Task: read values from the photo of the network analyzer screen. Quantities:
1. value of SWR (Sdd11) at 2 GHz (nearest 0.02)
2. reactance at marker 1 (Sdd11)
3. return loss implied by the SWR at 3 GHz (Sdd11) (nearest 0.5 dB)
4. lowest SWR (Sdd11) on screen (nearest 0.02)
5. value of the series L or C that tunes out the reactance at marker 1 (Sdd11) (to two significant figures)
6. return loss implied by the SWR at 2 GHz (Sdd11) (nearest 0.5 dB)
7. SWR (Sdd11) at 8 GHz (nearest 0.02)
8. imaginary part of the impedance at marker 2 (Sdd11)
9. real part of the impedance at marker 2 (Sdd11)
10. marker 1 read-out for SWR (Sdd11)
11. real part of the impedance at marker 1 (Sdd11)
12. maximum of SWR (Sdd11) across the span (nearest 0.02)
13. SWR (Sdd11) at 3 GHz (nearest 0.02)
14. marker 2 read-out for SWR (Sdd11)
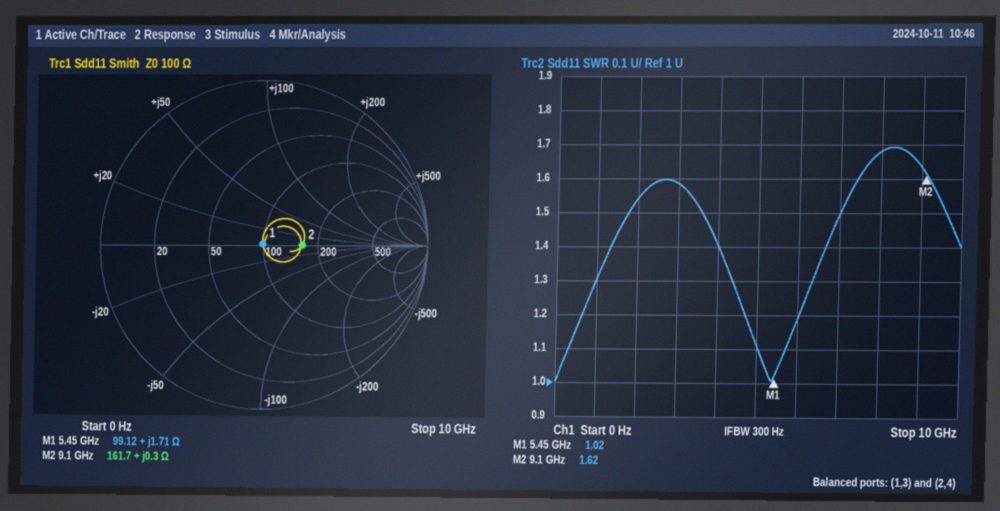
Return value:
1.54
+1.71 Ω
13.0 dB
1.00
17 pF
13.5 dB
1.68
+0.3 Ω
161.7 Ω
1.02
99.12 Ω
1.70
1.58
1.62
